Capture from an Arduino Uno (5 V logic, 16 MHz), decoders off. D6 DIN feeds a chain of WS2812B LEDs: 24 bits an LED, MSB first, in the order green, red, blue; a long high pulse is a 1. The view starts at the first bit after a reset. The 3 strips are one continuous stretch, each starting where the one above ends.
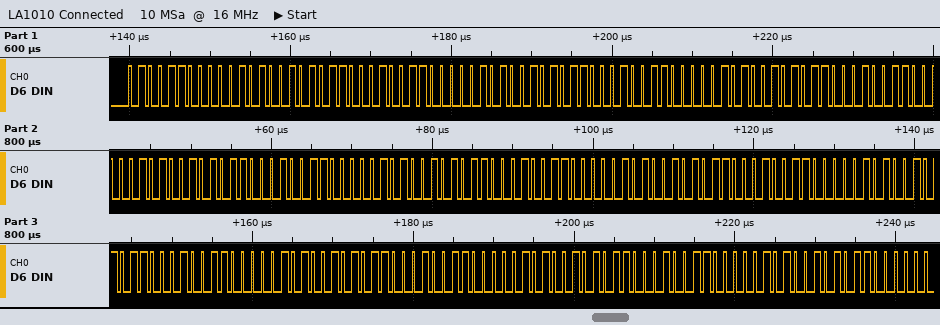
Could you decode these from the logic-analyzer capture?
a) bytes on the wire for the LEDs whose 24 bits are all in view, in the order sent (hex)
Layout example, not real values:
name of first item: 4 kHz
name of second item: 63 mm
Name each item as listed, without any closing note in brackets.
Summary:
bytes on the wire for the LEDs whose 24 bits are all in view, in the order sent: 4C 14 AC 4C 14 AC 4C 14 AC 4C 14 AC 4C 14 AC 4C 14 AC 4C 14 AC 4C 14 AC 4C 14 AC 4C 14 AC
